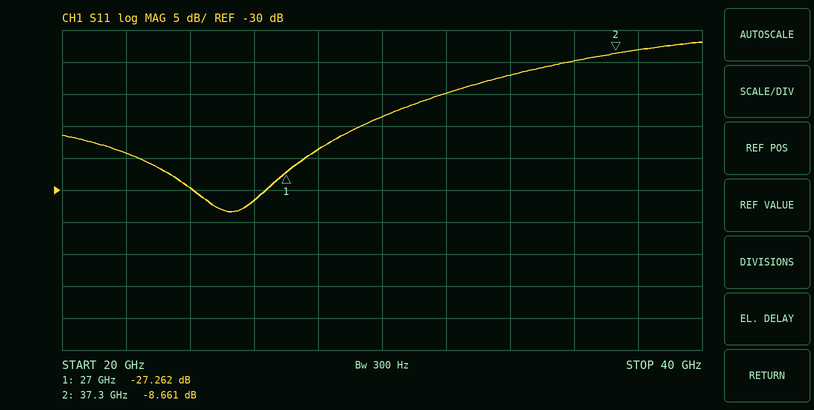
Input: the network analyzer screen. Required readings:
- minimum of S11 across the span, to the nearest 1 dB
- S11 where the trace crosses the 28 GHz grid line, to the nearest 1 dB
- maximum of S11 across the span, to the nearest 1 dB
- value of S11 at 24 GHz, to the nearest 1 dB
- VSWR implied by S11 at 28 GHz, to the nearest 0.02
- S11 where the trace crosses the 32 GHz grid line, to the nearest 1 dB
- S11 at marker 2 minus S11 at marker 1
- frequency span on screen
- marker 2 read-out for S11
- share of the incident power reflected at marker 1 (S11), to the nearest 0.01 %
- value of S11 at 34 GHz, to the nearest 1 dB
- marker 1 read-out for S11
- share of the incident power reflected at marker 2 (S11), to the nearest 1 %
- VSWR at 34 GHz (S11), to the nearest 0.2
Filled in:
-33 dB
-24 dB
-7 dB
-30 dB
1.14
-15 dB
18.601 dB
20 GHz
-8.661 dB
0.19 %
-12 dB
-27.262 dB
14 %
1.6
